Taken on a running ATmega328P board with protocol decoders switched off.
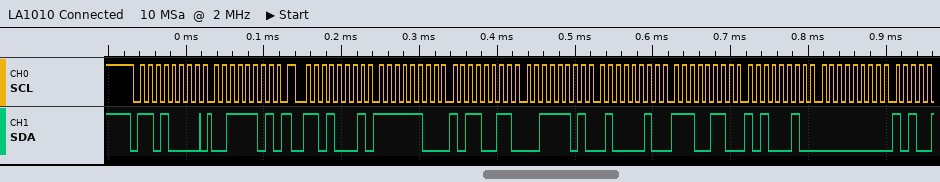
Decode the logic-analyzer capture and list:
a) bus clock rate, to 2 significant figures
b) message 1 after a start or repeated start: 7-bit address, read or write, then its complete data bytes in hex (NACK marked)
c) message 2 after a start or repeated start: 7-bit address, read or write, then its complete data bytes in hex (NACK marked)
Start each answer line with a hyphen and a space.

- 100 kHz
- 0x68 write: 3D
- 0x68 read: FC B3 3D 42 E6 A2 00
